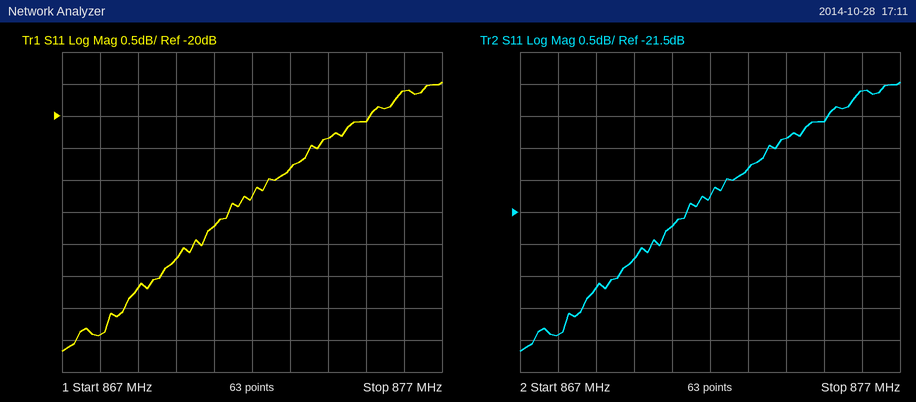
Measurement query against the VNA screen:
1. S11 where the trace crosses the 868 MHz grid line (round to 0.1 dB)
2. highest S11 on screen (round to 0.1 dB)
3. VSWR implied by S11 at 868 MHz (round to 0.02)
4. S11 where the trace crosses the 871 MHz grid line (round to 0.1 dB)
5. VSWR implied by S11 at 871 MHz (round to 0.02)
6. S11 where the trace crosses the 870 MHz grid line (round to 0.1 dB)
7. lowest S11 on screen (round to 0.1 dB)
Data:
-23.4 dB
-19.5 dB
1.14
-21.7 dB
1.18
-22.2 dB
-23.7 dB
